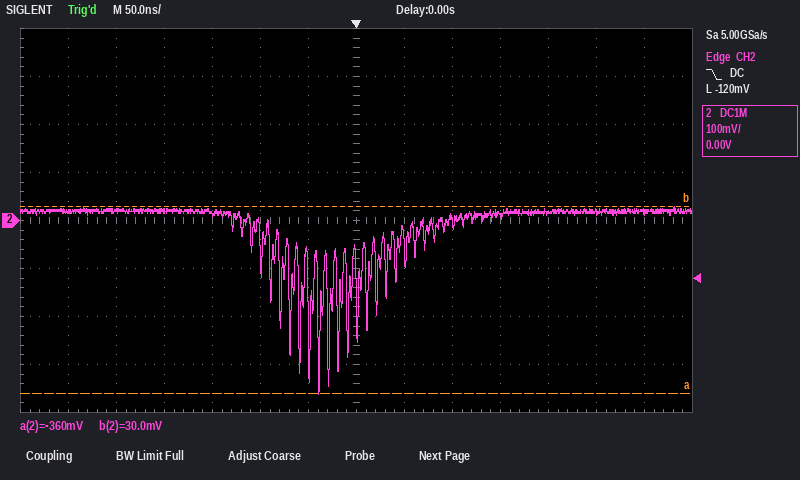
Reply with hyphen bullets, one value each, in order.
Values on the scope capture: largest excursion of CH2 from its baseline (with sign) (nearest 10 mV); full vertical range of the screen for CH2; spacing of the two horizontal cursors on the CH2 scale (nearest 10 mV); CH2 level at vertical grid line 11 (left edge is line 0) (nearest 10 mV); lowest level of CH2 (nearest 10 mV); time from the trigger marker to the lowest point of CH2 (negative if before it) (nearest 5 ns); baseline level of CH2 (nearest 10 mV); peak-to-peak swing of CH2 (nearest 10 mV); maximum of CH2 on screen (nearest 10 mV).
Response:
- -380 mV
- 800 mV
- 390 mV
- 10 mV
- -360 mV
- -40 ns
- 20 mV
- 390 mV
- 30 mV
